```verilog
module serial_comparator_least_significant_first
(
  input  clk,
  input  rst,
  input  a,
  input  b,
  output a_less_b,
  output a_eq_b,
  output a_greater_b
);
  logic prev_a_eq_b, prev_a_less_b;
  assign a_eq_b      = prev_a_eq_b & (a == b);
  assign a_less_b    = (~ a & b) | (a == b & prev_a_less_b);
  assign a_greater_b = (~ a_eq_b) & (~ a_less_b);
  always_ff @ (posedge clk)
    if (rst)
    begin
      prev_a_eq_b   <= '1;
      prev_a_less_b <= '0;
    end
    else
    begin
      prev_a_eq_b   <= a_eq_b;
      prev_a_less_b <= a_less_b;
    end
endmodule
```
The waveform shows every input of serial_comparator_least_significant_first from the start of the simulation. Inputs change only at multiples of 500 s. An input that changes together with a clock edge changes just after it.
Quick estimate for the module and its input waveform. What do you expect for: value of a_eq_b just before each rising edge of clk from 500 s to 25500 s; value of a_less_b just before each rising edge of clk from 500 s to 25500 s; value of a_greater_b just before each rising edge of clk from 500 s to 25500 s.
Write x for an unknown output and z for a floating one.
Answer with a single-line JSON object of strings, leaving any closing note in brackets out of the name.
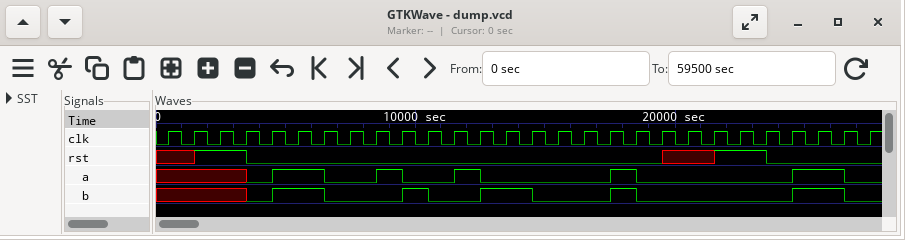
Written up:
{"value of a_eq_b just before each rising edge of clk from 500 s to 25500 s": "x x x x 1 1 1 1 1 0 0 0 0 0 0 0 0 0 0 0 0 0 0 1 1 1", "value of a_less_b just before each rising edge of clk from 500 s to 25500 s": "x x x x 0 0 0 0 0 0 1 1 0 1 1 1 1 1 1 1 1 1 1 0 0 0", "value of a_greater_b just before each rising edge of clk from 500 s to 25500 s": "x x x x 0 0 0 0 0 1 0 0 1 0 0 0 0 0 0 0 0 0 0 0 0 0"}
